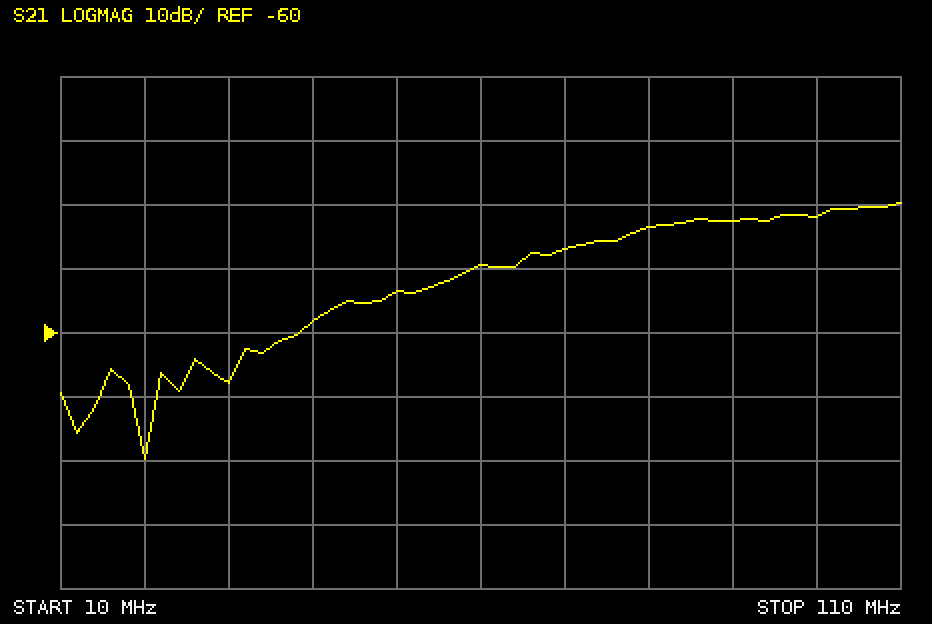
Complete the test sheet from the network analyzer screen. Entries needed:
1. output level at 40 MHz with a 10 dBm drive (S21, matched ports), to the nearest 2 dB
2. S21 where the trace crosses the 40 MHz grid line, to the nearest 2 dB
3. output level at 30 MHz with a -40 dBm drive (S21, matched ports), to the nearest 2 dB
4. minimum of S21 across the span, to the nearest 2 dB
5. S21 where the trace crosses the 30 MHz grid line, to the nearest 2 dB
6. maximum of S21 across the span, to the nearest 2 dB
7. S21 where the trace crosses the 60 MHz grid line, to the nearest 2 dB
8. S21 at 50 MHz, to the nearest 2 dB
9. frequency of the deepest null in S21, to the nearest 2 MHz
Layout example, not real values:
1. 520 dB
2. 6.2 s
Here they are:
1. -48 dBm
2. -58 dB
3. -108 dBm
4. -80 dB
5. -68 dB
6. -40 dB
7. -50 dB
8. -54 dB
9. 20 MHz
